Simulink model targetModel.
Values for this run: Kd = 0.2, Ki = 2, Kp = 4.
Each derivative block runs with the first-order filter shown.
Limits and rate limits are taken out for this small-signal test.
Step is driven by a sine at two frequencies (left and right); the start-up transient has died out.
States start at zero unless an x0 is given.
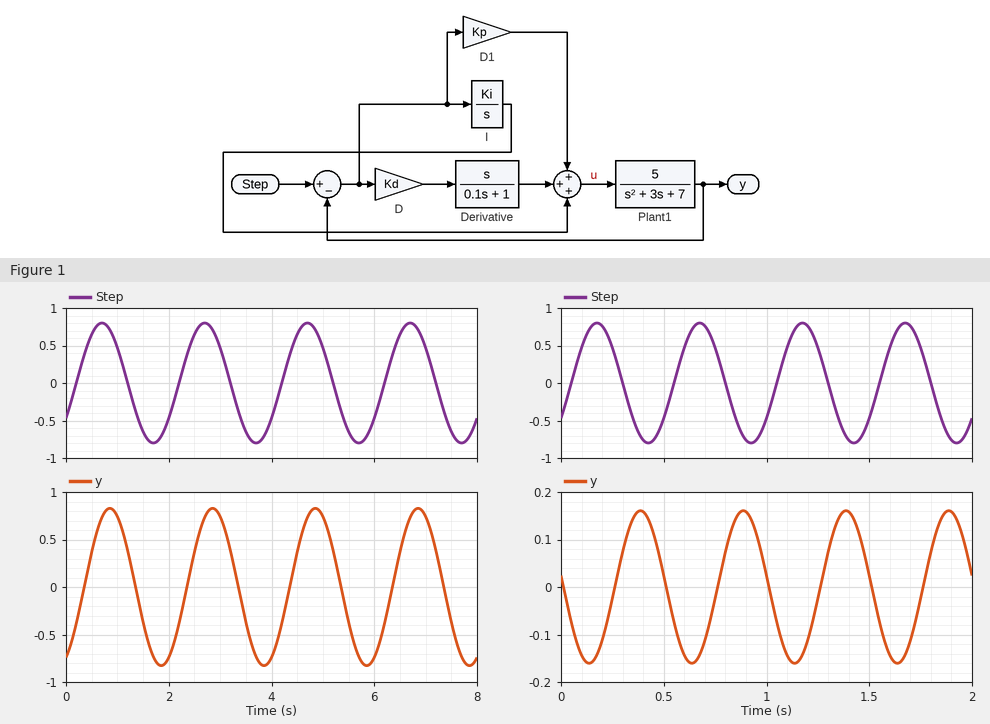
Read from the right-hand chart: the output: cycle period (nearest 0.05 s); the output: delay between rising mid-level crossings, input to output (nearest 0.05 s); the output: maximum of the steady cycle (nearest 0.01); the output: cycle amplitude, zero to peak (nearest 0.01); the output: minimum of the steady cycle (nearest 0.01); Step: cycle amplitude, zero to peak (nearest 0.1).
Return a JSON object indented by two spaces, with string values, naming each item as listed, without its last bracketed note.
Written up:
{
  "the output: cycle period": "0.50 s",
  "the output: delay between rising mid-level crossings, input to output": "0.20 s",
  "the output: maximum of the steady cycle": "0.16",
  "the output: cycle amplitude, zero to peak": "0.16",
  "the output: minimum of the steady cycle": "-0.16",
  "Step: cycle amplitude, zero to peak": "0.8"
}
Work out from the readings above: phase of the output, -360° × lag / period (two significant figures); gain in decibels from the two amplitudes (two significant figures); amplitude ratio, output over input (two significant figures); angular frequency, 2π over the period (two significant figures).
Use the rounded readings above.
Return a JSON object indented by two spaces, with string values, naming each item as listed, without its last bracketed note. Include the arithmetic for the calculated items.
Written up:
{
  "phase of the output, -360° × lag / period": "-360 × 0.2 / 0.5 = -140°",
  "gain in decibels from the two amplitudes": "20 log10(0.16 / 0.8) = -14 dB",
  "amplitude ratio, output over input": "0.16 / 0.8 = 0.20",
  "angular frequency, 2π over the period": "2π / 0.5 = 13 rad/s"
}
